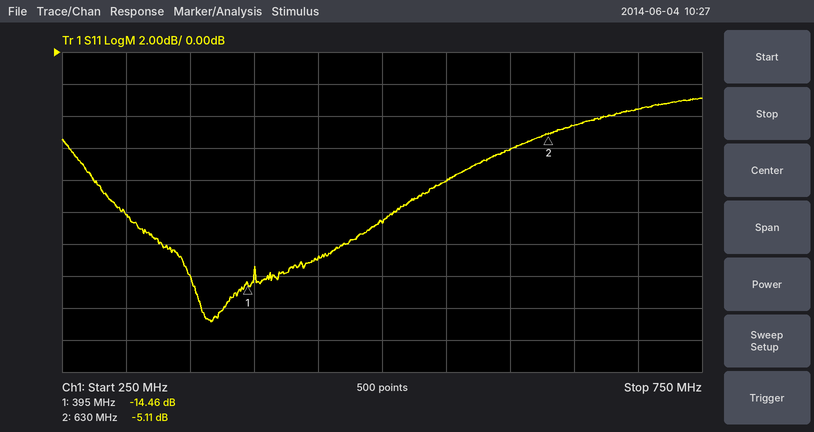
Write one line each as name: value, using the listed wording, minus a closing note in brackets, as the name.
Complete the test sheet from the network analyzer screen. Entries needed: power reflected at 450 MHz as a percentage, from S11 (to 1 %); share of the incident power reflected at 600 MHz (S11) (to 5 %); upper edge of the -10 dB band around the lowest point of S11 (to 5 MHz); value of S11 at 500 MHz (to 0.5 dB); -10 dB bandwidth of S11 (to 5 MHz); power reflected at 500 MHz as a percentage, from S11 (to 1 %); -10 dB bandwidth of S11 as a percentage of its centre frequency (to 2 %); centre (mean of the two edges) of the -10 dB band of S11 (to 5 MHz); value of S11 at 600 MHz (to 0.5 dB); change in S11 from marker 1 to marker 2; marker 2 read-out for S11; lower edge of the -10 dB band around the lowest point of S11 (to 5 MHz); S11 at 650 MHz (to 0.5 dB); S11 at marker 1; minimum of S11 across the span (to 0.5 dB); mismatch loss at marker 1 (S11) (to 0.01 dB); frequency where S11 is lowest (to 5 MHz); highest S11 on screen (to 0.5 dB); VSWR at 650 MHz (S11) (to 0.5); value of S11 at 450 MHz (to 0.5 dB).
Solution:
power reflected at 450 MHz as a percentage, from S11: 5 %
share of the incident power reflected at 600 MHz (S11): 25 %
upper edge of the -10 dB band around the lowest point of S11: 510 MHz
value of S11 at 500 MHz: -10.5 dB
-10 dB bandwidth of S11: 210 MHz
power reflected at 500 MHz as a percentage, from S11: 9 %
-10 dB bandwidth of S11 as a percentage of its centre frequency: 52 %
centre (mean of the two edges) of the -10 dB band of S11: 405 MHz
value of S11 at 600 MHz: -6.0 dB
change in S11 from marker 1 to marker 2: 9.35 dB
marker 2 read-out for S11: -5.11 dB
lower edge of the -10 dB band around the lowest point of S11: 300 MHz
S11 at 650 MHz: -4.5 dB
S11 at marker 1: -14.46 dB
minimum of S11 across the span: -17.0 dB
mismatch loss at marker 1 (S11): 0.16 dB
frequency where S11 is lowest: 365 MHz
highest S11 on screen: -3.0 dB
VSWR at 650 MHz (S11): 4.0
value of S11 at 450 MHz: -13.0 dB
